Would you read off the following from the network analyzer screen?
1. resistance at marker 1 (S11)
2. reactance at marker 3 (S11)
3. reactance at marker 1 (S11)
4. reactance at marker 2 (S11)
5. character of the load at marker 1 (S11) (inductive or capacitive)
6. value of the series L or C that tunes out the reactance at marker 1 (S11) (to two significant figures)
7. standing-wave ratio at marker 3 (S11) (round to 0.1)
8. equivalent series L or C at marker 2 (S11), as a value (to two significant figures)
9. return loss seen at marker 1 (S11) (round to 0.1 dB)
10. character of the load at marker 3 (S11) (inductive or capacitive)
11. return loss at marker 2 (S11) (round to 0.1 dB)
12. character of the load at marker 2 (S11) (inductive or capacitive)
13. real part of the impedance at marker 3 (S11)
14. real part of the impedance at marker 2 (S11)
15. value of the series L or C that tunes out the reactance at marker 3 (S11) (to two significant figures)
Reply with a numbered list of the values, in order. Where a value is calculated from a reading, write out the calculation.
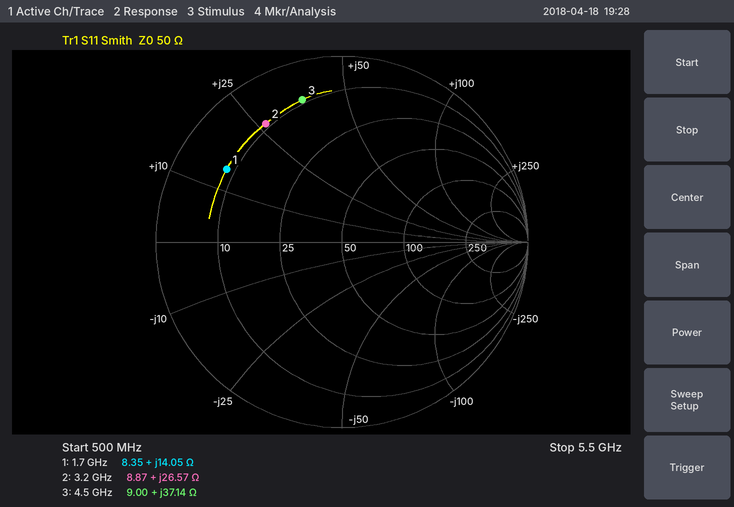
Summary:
1. 8.35 Ω
2. +37.14 Ω
3. +14.05 Ω
4. +26.57 Ω
5. inductive
6. C = 1/(2π × 1.7 GHz × 14.05 Ω) ≈ 6.7 pF
7. 8.7
8. L = 26.57 Ω/(2π × 3.2 GHz) ≈ 1.3 nH
9. 2.7 dB
10. inductive
11. 2.4 dB
12. inductive
13. 9.00 Ω
14. 8.87 Ω
15. C = 1/(2π × 4.5 GHz × 37.14 Ω) ≈ 952 fF, so 950 fF to two significant figures
